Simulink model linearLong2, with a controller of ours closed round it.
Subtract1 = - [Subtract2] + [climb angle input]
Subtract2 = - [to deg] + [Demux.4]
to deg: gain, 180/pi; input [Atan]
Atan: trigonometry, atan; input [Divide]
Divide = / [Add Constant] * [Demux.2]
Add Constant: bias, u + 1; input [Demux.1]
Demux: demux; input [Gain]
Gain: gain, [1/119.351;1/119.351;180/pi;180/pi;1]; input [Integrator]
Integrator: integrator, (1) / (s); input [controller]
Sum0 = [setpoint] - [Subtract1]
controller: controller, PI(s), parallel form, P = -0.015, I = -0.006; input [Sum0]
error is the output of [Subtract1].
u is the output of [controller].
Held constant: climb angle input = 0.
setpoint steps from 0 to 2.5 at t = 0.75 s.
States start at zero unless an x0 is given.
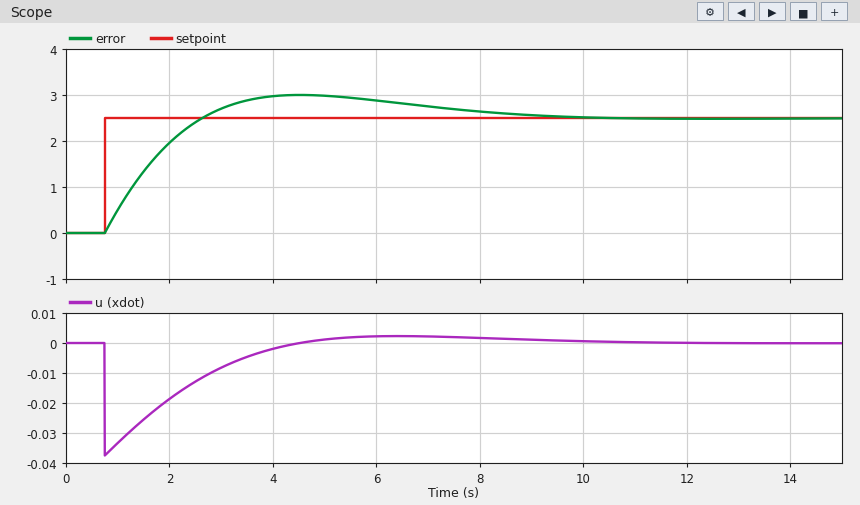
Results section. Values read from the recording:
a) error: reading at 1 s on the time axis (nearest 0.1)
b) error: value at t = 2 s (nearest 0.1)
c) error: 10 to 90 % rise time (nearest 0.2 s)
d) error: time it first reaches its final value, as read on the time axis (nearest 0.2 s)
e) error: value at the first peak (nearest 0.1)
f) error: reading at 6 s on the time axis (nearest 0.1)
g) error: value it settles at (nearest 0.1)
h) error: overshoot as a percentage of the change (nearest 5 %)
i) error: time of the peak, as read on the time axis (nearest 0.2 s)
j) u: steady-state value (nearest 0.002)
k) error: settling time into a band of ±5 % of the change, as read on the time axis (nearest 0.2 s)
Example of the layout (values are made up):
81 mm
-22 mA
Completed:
0.5
2.0
1.4 s
2.6 s
3.0
2.9
2.5
20 %
4.6 s
0.000
8.2 s
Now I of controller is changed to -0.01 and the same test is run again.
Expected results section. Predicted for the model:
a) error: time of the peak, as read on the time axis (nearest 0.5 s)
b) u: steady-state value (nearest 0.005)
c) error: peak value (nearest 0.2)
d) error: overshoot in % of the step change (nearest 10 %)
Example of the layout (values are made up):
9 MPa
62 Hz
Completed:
4.0 s
0.000
3.2
30 %
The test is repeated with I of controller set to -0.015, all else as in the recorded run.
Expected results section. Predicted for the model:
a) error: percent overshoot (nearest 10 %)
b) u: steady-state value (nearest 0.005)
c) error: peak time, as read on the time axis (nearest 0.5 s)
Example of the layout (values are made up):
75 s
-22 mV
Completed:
30 %
0.000
3.5 s
